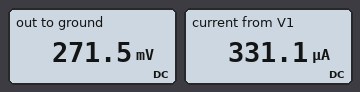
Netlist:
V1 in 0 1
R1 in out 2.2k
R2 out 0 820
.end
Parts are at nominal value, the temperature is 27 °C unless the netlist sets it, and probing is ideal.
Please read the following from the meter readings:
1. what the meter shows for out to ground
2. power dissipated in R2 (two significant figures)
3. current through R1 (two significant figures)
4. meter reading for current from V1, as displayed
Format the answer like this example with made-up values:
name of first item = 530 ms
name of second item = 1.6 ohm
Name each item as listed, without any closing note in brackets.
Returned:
what the meter shows for out to ground = 271.5 mV
power dissipated in R2 = 90 µW
current through R1 = 330 µA
meter reading for current from V1, as displayed = 331.1 µA
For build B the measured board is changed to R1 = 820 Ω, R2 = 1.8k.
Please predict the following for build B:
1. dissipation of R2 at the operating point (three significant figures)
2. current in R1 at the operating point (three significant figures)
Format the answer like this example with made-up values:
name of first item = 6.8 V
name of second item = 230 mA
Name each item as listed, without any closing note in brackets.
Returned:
dissipation of R2 at the operating point = 262 µW
current in R1 at the operating point = 382 µA
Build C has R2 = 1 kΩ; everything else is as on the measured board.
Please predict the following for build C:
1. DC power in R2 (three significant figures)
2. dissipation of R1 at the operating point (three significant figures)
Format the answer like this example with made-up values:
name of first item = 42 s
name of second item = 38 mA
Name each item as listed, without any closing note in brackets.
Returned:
DC power in R2 = 97.7 µW
dissipation of R1 at the operating point = 215 µW
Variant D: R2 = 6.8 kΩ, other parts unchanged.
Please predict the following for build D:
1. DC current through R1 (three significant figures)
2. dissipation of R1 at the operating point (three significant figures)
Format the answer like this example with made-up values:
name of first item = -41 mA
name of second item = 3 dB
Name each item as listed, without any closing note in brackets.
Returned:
DC current through R1 = 111 µA
dissipation of R1 at the operating point = 27.2 µW
